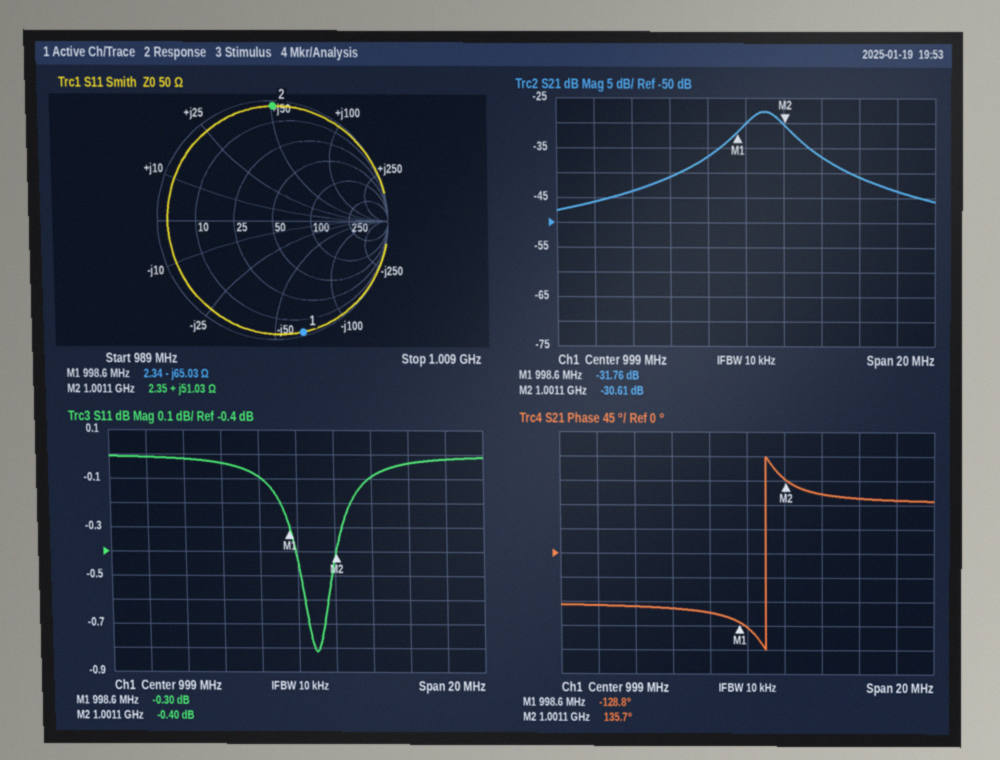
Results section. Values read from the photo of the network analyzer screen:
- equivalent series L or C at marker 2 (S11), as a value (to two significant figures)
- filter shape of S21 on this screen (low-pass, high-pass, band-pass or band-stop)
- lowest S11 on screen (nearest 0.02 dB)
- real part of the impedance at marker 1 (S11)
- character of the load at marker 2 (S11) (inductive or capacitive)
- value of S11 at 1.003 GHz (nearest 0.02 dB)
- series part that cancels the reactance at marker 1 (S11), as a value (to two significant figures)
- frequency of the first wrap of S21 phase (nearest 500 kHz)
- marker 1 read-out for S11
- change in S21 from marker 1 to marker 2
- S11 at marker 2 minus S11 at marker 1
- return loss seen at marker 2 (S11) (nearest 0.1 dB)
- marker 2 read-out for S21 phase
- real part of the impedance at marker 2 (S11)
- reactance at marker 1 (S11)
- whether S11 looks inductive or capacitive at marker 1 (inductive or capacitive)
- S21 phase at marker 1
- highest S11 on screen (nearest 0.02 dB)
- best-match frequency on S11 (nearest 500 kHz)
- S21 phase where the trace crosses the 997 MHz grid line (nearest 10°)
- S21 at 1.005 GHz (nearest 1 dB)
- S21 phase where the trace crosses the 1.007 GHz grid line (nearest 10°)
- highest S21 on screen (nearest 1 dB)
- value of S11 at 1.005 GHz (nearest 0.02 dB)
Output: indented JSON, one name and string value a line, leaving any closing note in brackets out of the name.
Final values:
{
  "equivalent series L or C at marker 2 (S11), as a value": "8.1 nH",
  "filter shape of S21 on this screen": "band-pass",
  "lowest S11 on screen": "-0.82 dB",
  "real part of the impedance at marker 1": "2.34 Ω",
  "character of the load at marker 2 (S11)": "inductive",
  "value of S11 at 1.003 GHz": "-0.10 dB",
  "series part that cancels the reactance at marker 1 (S11), as a value": "10 nH",
  "frequency of the first wrap of S21 phase": "1.0000 GHz",
  "marker 1 read-out for S11": "-0.30 dB",
  "change in S21 from marker 1 to marker 2": "1.15 dB",
  "S11 at marker 2 minus S11 at marker 1": "-0.10 dB",
  "return loss seen at marker 2 (S11)": "0.4 dB",
  "marker 2 read-out for S21 phase": "135.7°",
  "real part of the impedance at marker 2": "2.35 Ω",
  "reactance at marker 1": "-65.03 Ω",
  "whether S11 looks inductive or capacitive at marker 1": "capacitive",
  "S21 phase at marker 1": "-128.8°",
  "highest S11 on screen": "0.00 dB",
  "best-match frequency on S11": "1.0000 GHz",
  "S21 phase where the trace crosses the 997 MHz grid line": "-110°",
  "S21 at 1.005 GHz": "-41 dB",
  "S21 phase where the trace crosses the 1.007 GHz grid line": "100°",
  "highest S21 on screen": "-28 dB",
  "value of S11 at 1.005 GHz": "-0.04 dB"
}
